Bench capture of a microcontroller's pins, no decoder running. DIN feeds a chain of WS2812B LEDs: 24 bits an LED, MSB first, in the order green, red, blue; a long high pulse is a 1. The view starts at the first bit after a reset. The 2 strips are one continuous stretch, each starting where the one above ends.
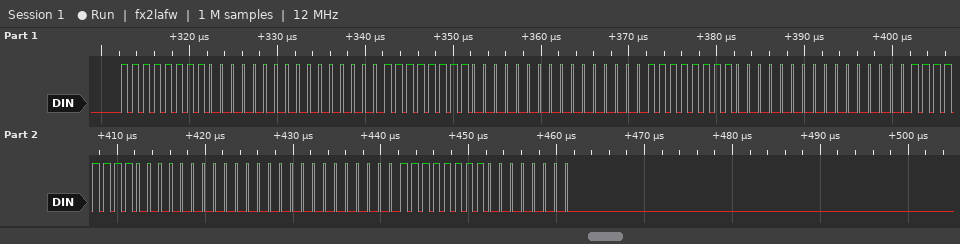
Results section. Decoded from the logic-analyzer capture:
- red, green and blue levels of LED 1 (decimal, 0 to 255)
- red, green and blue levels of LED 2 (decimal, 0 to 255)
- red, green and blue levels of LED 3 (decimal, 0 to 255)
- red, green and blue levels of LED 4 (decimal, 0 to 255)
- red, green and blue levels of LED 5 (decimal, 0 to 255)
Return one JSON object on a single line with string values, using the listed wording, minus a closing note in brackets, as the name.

{"red, green and blue levels of LED 1": "0, 255, 0", "red, green and blue levels of LED 2": "0, 255, 0", "red, green and blue levels of LED 3": "0, 255, 0", "red, green and blue levels of LED 4": "0, 255, 0", "red, green and blue levels of LED 5": "255, 0, 0"}
